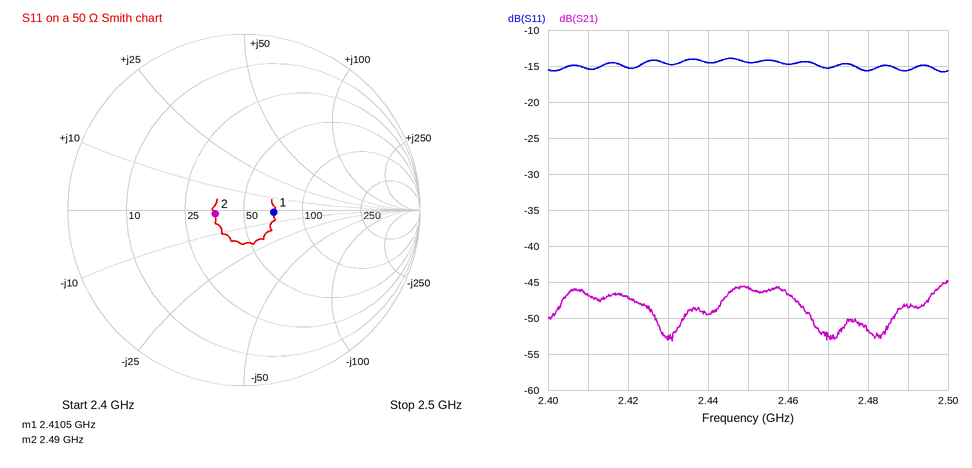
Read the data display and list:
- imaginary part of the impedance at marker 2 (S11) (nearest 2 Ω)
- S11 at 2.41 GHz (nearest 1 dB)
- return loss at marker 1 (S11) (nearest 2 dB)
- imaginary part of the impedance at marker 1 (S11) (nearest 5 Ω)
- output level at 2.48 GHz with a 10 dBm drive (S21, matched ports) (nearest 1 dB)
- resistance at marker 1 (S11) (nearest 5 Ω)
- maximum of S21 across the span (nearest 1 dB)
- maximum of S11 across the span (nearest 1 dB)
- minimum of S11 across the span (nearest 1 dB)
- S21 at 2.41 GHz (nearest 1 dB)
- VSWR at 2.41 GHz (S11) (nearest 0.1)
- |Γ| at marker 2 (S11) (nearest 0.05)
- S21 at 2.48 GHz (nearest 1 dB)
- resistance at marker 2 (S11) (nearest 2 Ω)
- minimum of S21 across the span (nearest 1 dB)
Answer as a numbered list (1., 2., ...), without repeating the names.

1. -2 Ω
2. -15 dB
3. 16 dB
4. 0 Ω
5. -42 dBm
6. 70 Ω
7. -45 dB
8. -14 dB
9. -16 dB
10. -47 dB
11. 1.4
12. 0.15
13. -52 dB
14. 36 Ω
15. -53 dB
